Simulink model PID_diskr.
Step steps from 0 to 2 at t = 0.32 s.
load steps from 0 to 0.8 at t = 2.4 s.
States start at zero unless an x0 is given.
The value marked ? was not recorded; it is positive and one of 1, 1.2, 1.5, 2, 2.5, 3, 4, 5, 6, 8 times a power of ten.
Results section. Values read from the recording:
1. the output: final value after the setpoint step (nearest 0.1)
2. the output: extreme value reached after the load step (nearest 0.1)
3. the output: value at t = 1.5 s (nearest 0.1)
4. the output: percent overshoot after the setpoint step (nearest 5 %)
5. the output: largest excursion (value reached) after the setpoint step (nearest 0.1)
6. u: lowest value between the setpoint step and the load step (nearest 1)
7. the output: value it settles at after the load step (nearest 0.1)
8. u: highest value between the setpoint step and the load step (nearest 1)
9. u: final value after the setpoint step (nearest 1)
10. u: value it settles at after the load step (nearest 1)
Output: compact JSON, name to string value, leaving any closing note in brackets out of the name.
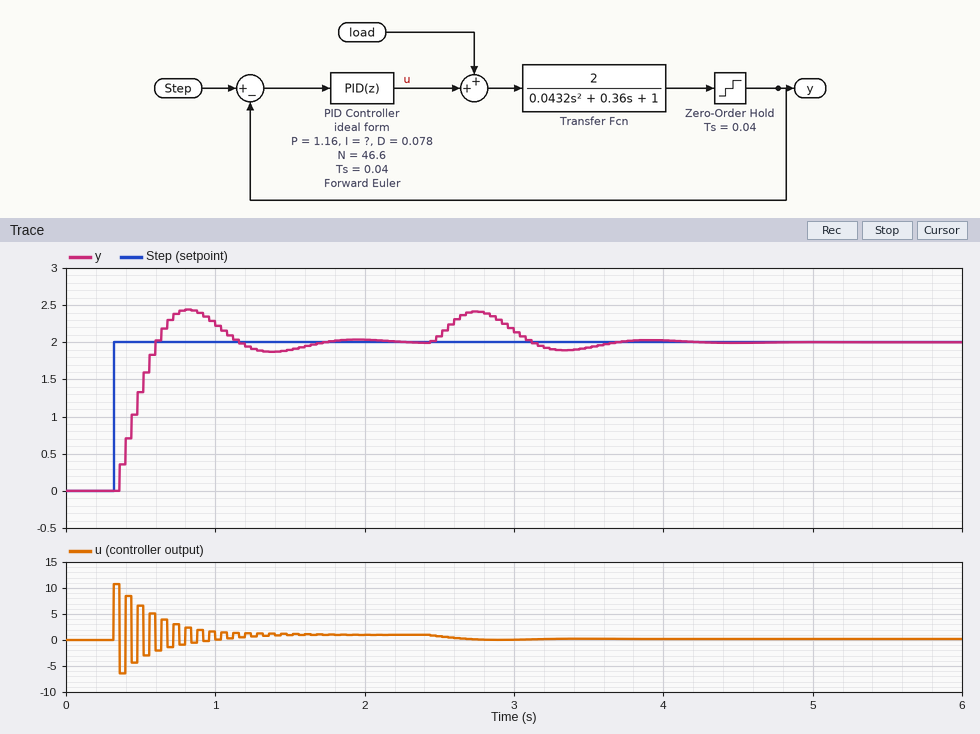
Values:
{"the output: final value after the setpoint step": "2.0", "the output: extreme value reached after the load step": "2.4", "the output: value at t = 1.5 s": "1.9", "the output: percent overshoot after the setpoint step": "20 %", "the output: largest excursion (value reached) after the setpoint step": "2.4", "u: lowest value between the setpoint step and the load step": "-6", "the output: value it settles at after the load step": "2.0", "u: highest value between the setpoint step and the load step": "11", "u: final value after the setpoint step": "1", "u: value it settles at after the load step": "0"}
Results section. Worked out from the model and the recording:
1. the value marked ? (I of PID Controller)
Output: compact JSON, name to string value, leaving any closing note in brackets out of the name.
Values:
{"the value marked ?": "5"}
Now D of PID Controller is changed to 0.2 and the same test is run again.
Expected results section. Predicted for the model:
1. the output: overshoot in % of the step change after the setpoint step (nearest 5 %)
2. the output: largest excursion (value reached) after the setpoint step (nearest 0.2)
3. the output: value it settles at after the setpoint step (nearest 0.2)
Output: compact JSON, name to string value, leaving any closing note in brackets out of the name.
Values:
{"the output: overshoot in % of the step change after the setpoint step": "10 %", "the output: largest excursion (value reached) after the setpoint step": "2.2", "the output: value it settles at after the setpoint step": "2.0"}
